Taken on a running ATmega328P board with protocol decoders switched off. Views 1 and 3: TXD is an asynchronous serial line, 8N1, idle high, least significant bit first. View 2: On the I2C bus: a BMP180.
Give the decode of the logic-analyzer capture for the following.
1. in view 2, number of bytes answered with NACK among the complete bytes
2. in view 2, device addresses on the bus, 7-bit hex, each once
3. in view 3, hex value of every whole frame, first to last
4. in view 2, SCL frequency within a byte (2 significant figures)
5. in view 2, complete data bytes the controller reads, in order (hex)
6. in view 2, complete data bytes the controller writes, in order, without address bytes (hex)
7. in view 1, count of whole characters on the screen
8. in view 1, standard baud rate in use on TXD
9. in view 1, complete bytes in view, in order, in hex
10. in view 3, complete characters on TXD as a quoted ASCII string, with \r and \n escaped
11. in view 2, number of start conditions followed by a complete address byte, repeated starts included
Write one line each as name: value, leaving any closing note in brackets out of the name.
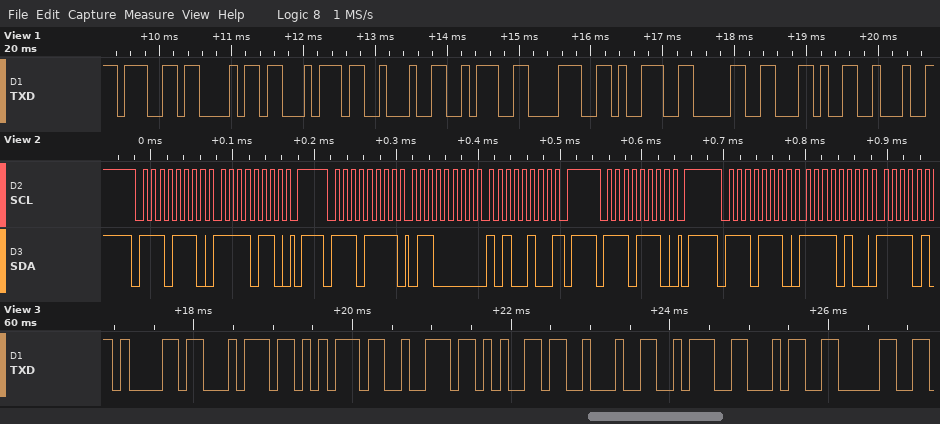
in view 2, number of bytes answered with NACK among the complete bytes: 1
in view 2, device addresses on the bus, 7-bit hex, each once: 0x77
in view 3, hex value of every whole frame, first to last: 61 74 75 72 65 22 3A 34 30
in view 2, SCL frequency within a byte: 100 kHz
in view 2, complete data bytes the controller reads, in order: 60 A4
in view 2, complete data bytes the controller writes, in order, without address bytes: F6 F4
in view 1, count of whole characters on the screen: 10
in view 1, standard baud rate in use on TXD: 9600 baud
in view 1, complete bytes in view, in order, in hex: 67 68 74 22 3A 38 39 30 2C 22
in view 3, complete characters on TXD as a quoted ASCII string, with \r and \n escaped: "ature\":40"
in view 2, number of start conditions followed by a complete address byte, repeated starts included: 4
